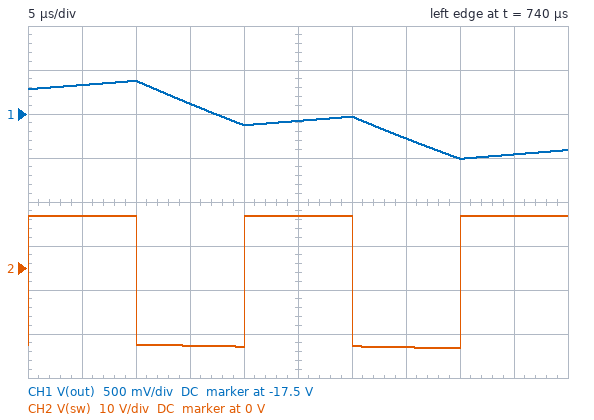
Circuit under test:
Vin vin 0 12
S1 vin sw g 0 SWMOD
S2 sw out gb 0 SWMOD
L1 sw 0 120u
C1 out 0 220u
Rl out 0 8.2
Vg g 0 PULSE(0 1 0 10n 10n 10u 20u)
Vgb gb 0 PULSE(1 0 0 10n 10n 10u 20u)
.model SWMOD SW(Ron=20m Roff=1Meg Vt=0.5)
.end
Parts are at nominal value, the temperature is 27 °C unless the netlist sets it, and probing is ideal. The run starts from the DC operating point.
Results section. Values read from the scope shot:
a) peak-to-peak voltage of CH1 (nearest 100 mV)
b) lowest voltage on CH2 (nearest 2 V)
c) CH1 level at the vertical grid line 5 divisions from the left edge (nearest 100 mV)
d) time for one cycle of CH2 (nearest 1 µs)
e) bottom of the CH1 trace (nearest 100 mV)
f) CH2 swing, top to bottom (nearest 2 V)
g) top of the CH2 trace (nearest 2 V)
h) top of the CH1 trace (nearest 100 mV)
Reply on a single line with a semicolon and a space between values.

900 mV; -18 V; -17.6 V; 20 µs; -18.0 V; 30 V; 12 V; -17.1 V
